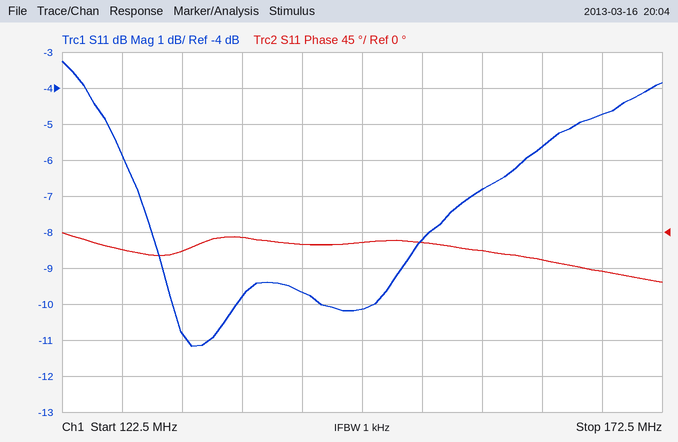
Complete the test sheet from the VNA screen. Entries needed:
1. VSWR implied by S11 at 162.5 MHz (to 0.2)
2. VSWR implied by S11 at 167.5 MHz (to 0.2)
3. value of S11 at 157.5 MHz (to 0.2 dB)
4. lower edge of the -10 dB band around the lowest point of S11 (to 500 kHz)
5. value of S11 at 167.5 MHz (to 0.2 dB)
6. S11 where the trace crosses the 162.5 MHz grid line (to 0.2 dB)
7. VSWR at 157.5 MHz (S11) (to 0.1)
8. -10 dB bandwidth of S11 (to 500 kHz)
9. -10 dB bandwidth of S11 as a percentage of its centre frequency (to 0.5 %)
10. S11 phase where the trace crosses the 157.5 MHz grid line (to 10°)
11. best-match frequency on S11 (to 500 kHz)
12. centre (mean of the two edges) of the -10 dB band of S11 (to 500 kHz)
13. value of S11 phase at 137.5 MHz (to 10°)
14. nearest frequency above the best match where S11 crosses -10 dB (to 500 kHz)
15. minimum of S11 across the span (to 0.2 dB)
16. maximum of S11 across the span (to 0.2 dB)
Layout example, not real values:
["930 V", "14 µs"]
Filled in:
["3.2", "3.8", "-6.8 dB", "131.5 MHz", "-4.8 dB", "-5.6 dB", "2.7", "5.5 MHz", "4.0 %", "-20°", "133.5 MHz", "134.5 MHz", "-10°", "137.0 MHz", "-11.2 dB", "-3.2 dB"]
